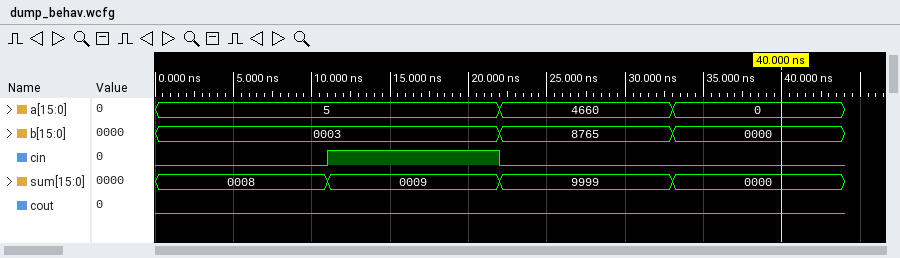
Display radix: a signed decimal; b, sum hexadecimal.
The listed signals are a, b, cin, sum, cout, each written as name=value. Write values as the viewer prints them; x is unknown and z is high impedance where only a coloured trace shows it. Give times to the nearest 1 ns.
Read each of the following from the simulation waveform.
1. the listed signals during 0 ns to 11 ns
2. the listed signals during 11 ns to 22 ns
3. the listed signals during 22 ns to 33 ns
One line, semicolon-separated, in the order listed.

a=5, b=0003, cin=0, sum=0008, cout=0; a=5, b=0003, cin=1, sum=0009, cout=0; a=4660, b=8765, cin=0, sum=9999, cout=0
